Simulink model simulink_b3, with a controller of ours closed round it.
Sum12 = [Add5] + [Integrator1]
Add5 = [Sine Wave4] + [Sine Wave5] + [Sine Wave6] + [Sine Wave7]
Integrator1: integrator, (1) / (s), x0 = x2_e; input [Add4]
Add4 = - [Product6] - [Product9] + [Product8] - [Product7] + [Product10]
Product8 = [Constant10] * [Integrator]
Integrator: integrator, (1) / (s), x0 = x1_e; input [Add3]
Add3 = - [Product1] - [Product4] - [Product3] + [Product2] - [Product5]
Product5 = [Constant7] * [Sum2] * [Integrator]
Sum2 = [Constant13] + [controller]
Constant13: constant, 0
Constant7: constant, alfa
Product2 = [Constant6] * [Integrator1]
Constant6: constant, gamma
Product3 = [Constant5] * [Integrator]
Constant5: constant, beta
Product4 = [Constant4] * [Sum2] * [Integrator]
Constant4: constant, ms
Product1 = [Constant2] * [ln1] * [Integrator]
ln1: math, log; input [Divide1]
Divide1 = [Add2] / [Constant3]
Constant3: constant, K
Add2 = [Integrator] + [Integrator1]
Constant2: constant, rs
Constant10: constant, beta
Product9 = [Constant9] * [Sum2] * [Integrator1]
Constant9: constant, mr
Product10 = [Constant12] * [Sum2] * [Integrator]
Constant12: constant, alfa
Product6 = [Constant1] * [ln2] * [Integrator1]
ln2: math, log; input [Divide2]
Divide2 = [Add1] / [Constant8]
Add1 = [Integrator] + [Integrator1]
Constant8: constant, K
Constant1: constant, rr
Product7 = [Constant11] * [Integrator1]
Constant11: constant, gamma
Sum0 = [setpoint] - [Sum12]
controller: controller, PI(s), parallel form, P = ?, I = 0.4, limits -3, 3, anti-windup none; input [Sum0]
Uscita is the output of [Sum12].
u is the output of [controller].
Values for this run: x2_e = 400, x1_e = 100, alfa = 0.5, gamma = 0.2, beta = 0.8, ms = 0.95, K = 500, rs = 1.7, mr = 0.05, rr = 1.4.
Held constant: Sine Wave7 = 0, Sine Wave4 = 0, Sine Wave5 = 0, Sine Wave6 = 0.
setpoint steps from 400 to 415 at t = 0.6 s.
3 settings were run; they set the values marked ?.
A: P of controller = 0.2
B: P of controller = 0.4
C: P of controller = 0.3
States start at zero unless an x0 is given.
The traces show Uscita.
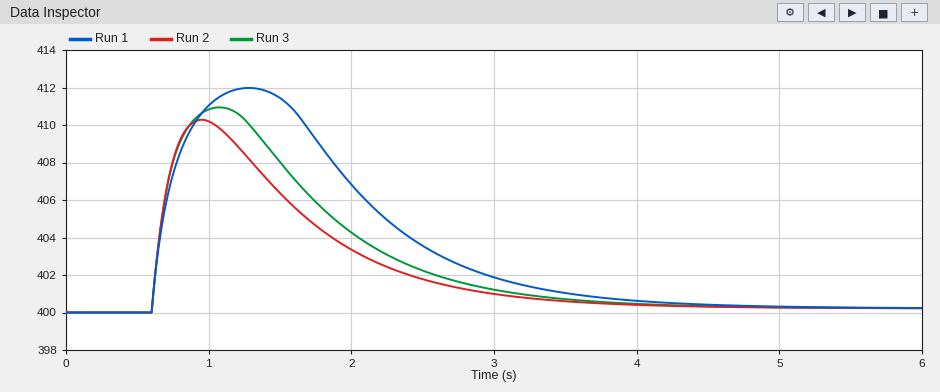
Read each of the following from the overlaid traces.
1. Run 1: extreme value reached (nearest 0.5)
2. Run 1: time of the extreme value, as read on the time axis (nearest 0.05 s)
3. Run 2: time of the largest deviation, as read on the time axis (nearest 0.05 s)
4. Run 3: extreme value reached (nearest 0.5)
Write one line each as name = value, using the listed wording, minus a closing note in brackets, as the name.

Run 1: extreme value reached = 412.0
Run 1: time of the extreme value, as read on the time axis = 1.30 s
Run 2: time of the largest deviation, as read on the time axis = 0.95 s
Run 3: extreme value reached = 411.0
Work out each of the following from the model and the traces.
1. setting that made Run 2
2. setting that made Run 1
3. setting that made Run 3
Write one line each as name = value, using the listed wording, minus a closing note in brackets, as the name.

setting that made Run 2 = B
setting that made Run 1 = A
setting that made Run 3 = C
